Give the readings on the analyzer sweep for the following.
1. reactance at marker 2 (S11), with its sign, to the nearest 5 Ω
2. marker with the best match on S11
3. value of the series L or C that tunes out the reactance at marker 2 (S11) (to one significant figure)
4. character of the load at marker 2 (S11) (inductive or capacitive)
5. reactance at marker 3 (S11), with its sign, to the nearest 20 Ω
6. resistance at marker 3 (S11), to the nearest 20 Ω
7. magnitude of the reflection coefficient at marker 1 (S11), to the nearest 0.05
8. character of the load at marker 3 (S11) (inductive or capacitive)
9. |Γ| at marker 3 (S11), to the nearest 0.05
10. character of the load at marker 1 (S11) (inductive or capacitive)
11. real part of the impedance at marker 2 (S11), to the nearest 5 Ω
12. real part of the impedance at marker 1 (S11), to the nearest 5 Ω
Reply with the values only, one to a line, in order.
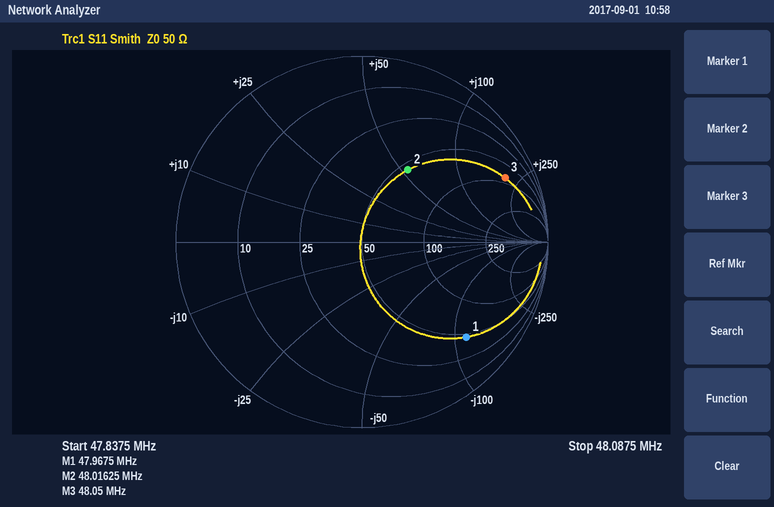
+55 Ω
marker 2
60 pF
inductive
+200 Ω
80 Ω
0.75
inductive
0.85
capacitive
55 Ω
45 Ω
